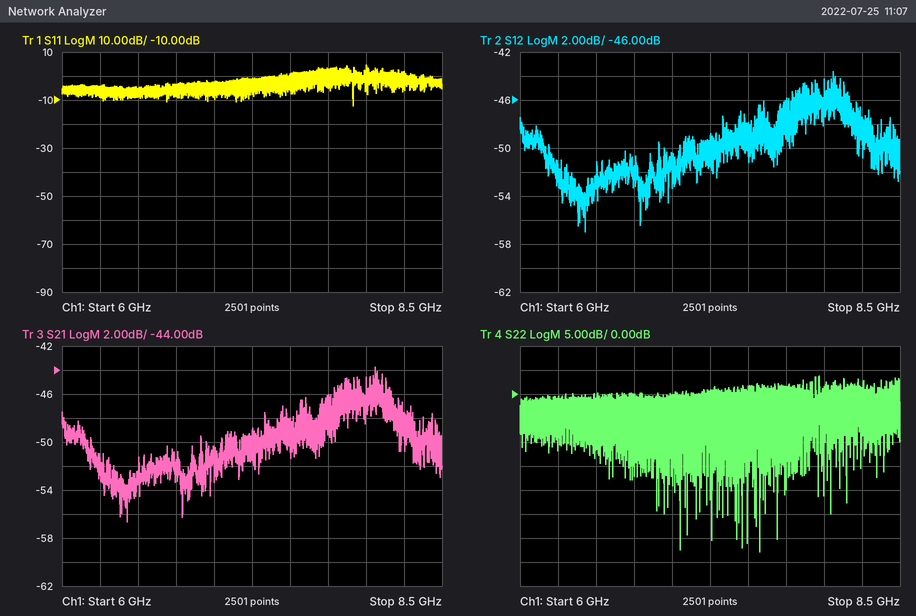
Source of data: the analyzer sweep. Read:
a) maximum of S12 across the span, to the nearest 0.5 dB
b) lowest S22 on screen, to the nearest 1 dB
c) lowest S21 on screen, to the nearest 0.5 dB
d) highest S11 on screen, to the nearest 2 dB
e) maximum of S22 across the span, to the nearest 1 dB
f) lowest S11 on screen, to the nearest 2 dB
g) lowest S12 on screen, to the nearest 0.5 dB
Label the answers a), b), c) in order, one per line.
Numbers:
a) -43.5 dB
b) -33 dB
c) -56.5 dB
d) 4 dB
e) 4 dB
f) -12 dB
g) -57.0 dB
